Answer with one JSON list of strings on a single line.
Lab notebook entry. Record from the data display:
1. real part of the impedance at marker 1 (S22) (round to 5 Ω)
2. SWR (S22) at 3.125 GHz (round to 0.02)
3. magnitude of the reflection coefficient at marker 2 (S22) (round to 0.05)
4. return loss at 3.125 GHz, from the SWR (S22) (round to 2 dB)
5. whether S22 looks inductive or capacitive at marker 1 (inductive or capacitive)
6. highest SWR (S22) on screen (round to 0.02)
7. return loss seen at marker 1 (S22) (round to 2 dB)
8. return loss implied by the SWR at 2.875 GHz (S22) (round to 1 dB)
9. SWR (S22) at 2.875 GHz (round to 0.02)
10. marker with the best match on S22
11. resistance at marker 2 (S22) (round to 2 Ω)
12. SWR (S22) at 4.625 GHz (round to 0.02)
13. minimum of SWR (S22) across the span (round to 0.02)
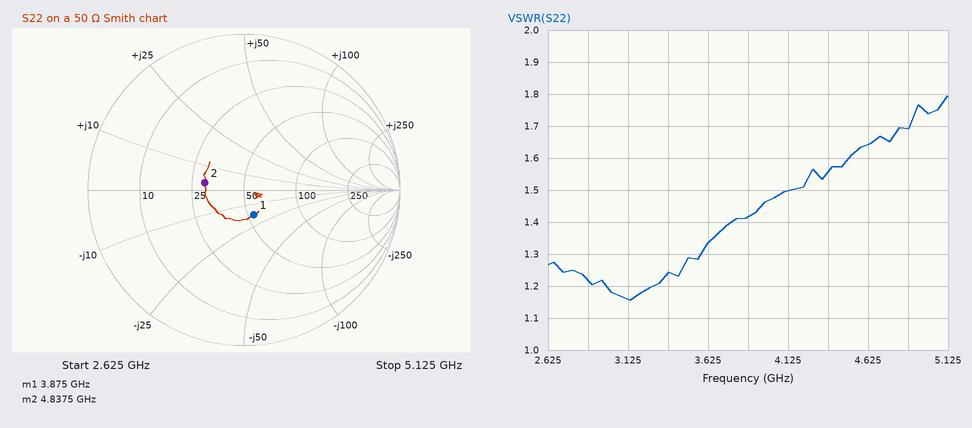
["55 Ω", "1.16", "0.25", "22 dB", "capacitive", "1.80", "16 dB", "20 dB", "1.22", "marker 1", "30 Ω", "1.64", "1.16"]
